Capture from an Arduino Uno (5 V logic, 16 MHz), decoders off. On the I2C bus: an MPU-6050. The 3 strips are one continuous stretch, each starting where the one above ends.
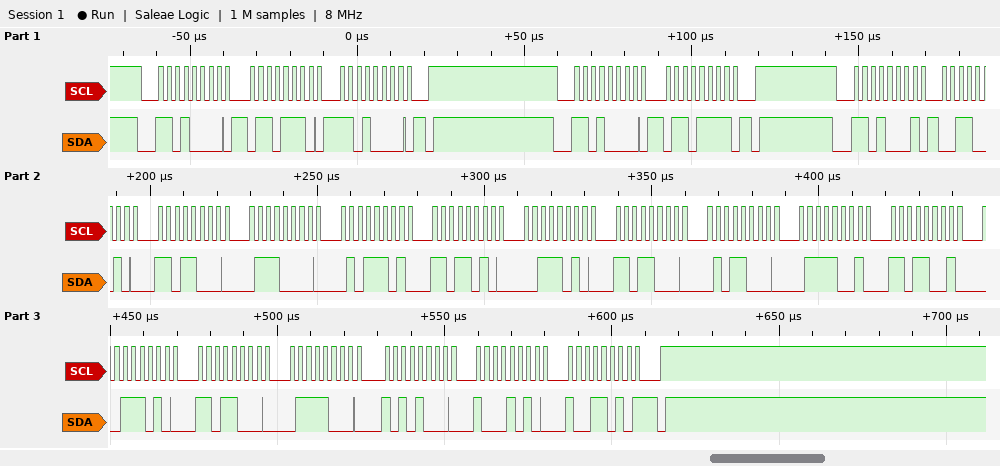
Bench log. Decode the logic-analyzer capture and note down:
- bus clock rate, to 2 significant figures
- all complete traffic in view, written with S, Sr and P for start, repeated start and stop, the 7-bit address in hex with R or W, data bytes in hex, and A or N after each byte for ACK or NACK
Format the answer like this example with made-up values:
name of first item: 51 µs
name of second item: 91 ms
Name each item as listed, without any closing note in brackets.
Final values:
bus clock rate, to 2 significant figures: 400 kHz
all complete traffic in view, written with S, Sr and P for start, repeated start and stop, the 7-bit address in hex with R or W, data bytes in hex, and A or N after each byte for ACK or NACK: S 68W A 6E A D0 A P S 68W A 6F A P S 68R A 32 A D8 A 70 A 5D A DA A 3A A D8 A 58 A 79 A D9 A 3A A D8 A 78 A A8 A 8A A 9A N P
